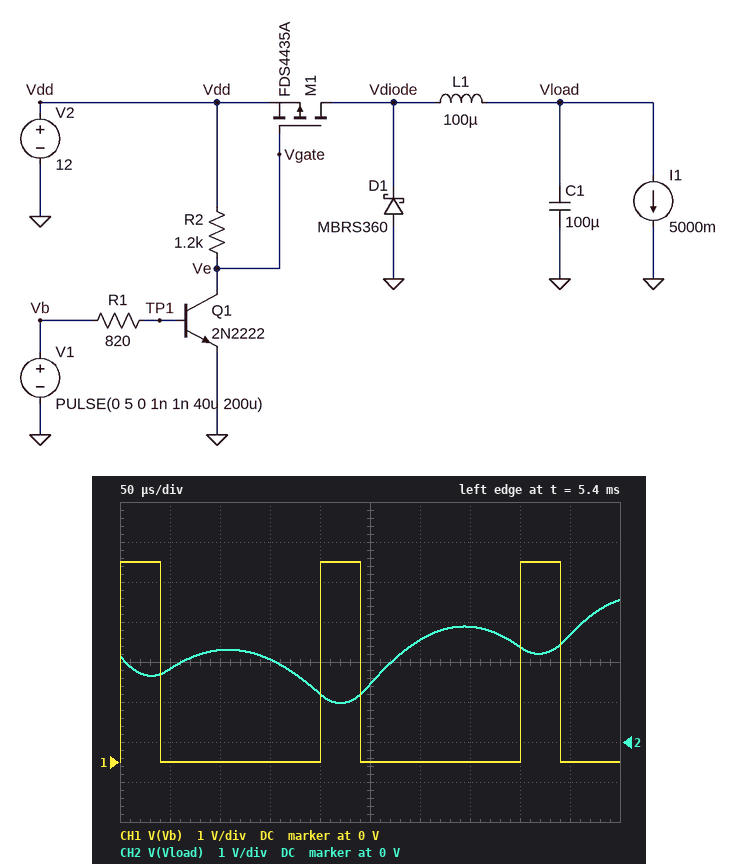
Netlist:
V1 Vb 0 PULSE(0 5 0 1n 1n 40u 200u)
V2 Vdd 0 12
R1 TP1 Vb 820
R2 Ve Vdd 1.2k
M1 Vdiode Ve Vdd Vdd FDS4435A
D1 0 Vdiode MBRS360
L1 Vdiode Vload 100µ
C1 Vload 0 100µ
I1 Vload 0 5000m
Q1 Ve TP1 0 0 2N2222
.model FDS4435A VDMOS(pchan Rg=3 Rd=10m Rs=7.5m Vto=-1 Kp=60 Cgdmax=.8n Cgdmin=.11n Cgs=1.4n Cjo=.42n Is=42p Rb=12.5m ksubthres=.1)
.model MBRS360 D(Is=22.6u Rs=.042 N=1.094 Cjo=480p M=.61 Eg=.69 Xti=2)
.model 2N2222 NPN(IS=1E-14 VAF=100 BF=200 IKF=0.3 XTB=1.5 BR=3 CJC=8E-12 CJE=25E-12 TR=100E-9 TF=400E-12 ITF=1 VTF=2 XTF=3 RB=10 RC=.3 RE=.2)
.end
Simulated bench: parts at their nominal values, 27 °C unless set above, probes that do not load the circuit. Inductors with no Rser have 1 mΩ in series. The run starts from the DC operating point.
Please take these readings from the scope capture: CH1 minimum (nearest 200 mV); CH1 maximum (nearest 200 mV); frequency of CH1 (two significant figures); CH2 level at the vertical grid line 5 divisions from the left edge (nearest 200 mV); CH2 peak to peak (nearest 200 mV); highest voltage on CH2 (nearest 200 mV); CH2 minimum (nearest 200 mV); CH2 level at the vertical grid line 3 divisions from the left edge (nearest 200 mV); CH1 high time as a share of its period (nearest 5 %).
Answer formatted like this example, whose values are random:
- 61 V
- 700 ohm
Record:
- 0 V
- 5.0 V
- 5.0 kHz
- 1.4 V
- 2.6 V
- 3.6 V
- 1.0 V
- 2.0 V
- 20 %
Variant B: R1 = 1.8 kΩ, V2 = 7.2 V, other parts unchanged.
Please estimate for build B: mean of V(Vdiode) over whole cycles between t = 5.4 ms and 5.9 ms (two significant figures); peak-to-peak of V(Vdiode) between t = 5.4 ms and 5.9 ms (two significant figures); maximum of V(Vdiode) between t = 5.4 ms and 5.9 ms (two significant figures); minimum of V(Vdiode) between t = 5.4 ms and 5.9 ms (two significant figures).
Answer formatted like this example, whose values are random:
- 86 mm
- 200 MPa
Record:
- 1.2 V
- 7.8 V
- 7.1 V
- -640 mV
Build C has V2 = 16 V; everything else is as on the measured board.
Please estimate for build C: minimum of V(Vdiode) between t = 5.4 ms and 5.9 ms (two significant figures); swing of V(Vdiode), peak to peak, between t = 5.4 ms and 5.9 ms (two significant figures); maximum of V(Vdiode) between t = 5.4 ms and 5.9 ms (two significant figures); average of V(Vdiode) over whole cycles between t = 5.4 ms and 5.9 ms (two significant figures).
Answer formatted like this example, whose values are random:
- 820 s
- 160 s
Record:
- -720 mV
- 17 V
- 16 V
- 3.4 V
